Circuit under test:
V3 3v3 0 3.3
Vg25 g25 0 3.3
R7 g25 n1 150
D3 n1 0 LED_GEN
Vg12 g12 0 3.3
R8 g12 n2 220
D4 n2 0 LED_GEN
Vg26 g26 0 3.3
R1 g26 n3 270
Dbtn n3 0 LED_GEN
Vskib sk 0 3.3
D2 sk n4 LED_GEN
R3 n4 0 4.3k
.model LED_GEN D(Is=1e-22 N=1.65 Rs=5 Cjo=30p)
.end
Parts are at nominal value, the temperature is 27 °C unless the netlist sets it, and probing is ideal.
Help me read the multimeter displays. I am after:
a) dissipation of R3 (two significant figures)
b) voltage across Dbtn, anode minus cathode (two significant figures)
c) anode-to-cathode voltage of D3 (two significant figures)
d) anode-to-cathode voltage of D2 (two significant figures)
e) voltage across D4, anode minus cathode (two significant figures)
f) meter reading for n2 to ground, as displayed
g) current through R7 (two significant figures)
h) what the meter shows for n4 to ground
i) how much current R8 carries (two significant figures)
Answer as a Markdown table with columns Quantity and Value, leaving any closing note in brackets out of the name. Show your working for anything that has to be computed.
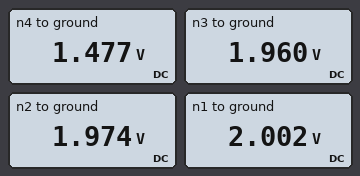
| Quantity | Value |
|---|---|
| dissipation of R3 | (1.477 V)^2 / 4.3 kΩ = 510 µW |
| voltage across Dbtn, anode minus cathode | 1.96 V = 2.0 V |
| anode-to-cathode voltage of D3 | 2.002 V = 2.0 V |
| anode-to-cathode voltage of D2 | 3.3 V - 1.477 V = 1.8 V |
| voltage across D4, anode minus cathode | 1.974 V = 2.0 V |
| meter reading for n2 to ground, as displayed | 1.974 V |
| current through R7 | (3.3 V - 2.002 V) / 150 Ω = 8.7 mA |
| what the meter shows for n4 to ground | 1.477 V |
| how much current R8 carries | (3.3 V - 1.974 V) / 220 Ω = 6.0 mA |
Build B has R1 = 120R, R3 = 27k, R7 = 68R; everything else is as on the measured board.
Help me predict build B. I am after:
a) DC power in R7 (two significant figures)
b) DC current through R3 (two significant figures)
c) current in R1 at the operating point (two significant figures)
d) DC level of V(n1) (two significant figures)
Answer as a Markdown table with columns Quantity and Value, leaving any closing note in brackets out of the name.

| Quantity | Value |
|---|---|
| DC power in R7 | 22 mW |
| DC current through R3 | 58 µA |
| current in R1 at the operating point | 11 mA |
| DC level of V(n1) | 2.1 V |
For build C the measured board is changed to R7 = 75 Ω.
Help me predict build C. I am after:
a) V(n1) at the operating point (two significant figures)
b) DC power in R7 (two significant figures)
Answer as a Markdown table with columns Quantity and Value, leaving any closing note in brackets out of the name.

| Quantity | Value |
|---|---|
| V(n1) at the operating point | 2.1 V |
| DC power in R7 | 20 mW |
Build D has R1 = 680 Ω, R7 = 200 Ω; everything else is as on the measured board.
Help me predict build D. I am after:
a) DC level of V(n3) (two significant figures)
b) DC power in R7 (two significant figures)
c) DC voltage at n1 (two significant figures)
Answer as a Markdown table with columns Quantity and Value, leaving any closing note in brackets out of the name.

| Quantity | Value |
|---|---|
| DC level of V(n3) | 1.9 V |
| DC power in R7 | 8.7 mW |
| DC voltage at n1 | 2.0 V |
